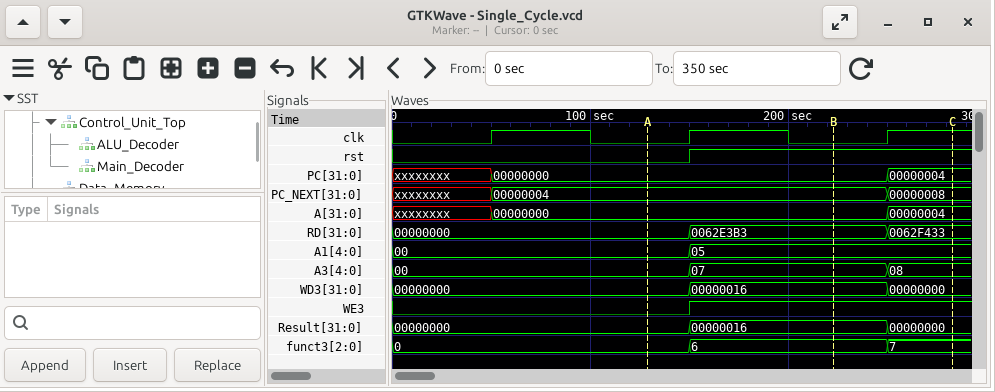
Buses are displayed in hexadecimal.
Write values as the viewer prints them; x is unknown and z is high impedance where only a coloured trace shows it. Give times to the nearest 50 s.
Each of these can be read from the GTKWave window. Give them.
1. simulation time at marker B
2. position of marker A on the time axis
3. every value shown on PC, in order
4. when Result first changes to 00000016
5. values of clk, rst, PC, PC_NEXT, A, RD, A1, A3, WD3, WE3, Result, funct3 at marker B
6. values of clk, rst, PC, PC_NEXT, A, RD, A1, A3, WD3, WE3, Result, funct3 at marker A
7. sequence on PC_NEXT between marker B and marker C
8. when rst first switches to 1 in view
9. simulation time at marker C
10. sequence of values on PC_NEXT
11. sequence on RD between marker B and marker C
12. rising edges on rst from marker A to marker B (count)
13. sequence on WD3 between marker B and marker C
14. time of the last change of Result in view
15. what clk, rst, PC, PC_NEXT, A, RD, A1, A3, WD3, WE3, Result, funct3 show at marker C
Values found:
200 s
150 s
xxxxxxxx, 00000000, 00000004
150 s
clk=0, rst=1, PC=00000000, PC_NEXT=00000004, A=00000000, RD=0062E3B3, A1=05, A3=07, WD3=00000016, WE3=1, Result=00000016, funct3=6
clk=0, rst=0, PC=00000000, PC_NEXT=00000004, A=00000000, RD=00000000, A1=00, A3=00, WD3=00000000, WE3=0, Result=00000000, funct3=0
00000004, 00000008
150 s
300 s
xxxxxxxx, 00000004, 00000008
0062E3B3, 0062F433
1
00000016, 00000000
250 s
clk=1, rst=1, PC=00000004, PC_NEXT=00000008, A=00000004, RD=0062F433, A1=05, A3=08, WD3=00000000, WE3=1, Result=00000000, funct3=7
